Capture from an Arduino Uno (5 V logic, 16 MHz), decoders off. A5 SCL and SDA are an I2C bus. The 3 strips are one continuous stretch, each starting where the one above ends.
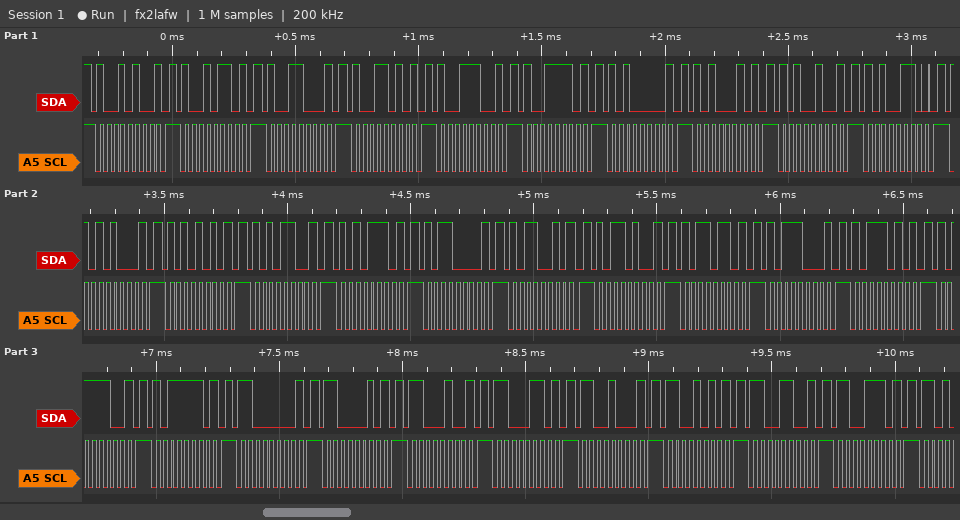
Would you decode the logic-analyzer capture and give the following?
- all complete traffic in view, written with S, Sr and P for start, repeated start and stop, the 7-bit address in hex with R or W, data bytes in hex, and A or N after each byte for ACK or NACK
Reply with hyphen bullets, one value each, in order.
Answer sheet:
- S 4AW N P S 4BW N P S 4CW N P S 4DW N P S 4EW N P S 4FW N P S 50W N P S 51W N P S 52W N P S 53W A P S 54W N P S 55W N P S 56W N P S 57W N P S 58W N P S 59W N P S 5AW N P S 5BW N P S 5CW N P S 5DW N P S 5EW N P S 5FW N P S 60W N P S 61W N P S 62W N P S 63W N P S 64W N P S 65W N P S 66W N P S 67W N P
